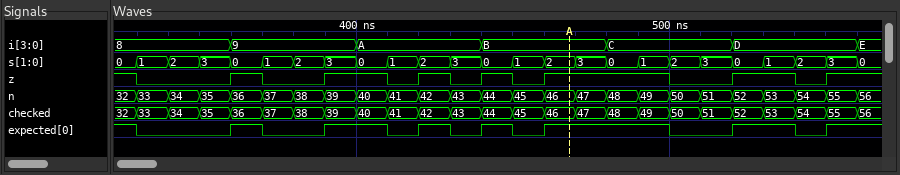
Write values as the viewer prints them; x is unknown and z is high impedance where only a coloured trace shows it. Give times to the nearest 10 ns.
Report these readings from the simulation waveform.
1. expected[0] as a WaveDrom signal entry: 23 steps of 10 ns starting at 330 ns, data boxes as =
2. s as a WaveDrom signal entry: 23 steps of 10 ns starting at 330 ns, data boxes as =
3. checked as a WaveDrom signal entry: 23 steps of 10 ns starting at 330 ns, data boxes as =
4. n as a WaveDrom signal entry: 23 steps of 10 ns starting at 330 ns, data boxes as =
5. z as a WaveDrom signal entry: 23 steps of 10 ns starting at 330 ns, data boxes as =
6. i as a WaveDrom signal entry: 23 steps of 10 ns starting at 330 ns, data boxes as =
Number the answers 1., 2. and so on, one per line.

1. {name: 'expected[0]', wave: '0..10.1.010101...0.1.01'}
2. {name: 's', wave: '=======================', data: '1 2 3 0 1 2 3 0 1 2 3 0 1 2 3 0 1 2 3 0 1 2 3'}
3. {name: 'checked', wave: '=======================', data: '33 34 35 36 37 38 39 40 41 42 43 44 45 46 47 48 49 50 51 52 53 54 55'}
4. {name: 'n', wave: '=======================', data: '33 34 35 36 37 38 39 40 41 42 43 44 45 46 47 48 49 50 51 52 53 54 55'}
5. {name: 'z', wave: '0..10.1.010101...0.1.01'}
6. {name: 'i', wave: '=..=...=...=...=...=...', data: '8 9 A B C D'}
